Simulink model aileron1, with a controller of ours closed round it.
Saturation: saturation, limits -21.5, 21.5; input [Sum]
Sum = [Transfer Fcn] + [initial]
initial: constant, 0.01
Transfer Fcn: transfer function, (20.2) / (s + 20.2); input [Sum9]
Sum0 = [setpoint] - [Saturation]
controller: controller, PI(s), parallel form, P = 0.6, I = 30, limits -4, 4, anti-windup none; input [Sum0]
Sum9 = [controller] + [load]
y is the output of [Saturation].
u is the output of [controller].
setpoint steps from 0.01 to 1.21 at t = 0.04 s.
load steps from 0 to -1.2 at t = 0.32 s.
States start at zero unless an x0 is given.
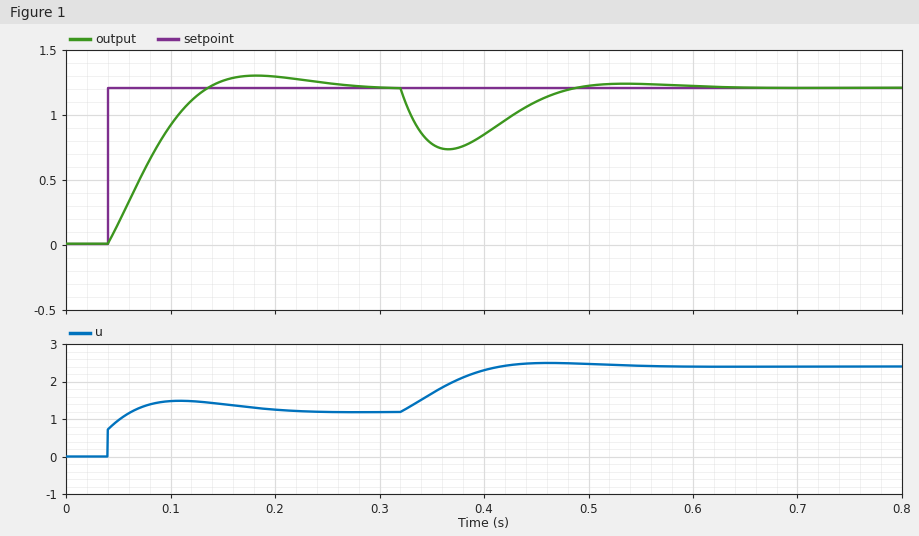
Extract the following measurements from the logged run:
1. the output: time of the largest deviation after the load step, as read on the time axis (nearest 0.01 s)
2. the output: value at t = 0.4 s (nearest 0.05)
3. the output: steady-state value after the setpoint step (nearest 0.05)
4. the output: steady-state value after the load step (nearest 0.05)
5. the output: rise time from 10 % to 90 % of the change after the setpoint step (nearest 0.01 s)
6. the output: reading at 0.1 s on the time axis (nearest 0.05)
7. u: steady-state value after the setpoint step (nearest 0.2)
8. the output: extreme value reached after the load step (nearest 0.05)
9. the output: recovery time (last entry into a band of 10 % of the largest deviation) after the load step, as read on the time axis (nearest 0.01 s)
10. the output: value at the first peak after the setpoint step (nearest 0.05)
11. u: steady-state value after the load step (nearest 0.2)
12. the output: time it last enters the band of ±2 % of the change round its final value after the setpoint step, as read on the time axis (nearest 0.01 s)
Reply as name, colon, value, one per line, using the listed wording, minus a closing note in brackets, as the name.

the output: time of the largest deviation after the load step, as read on the time axis: 0.37 s
the output: value at t = 0.4 s: 0.85
the output: steady-state value after the setpoint step: 1.20
the output: steady-state value after the load step: 1.20
the output: rise time from 10 % to 90 % of the change after the setpoint step: 0.07 s
the output: reading at 0.1 s on the time axis: 0.90
u: steady-state value after the setpoint step: 1.2
the output: extreme value reached after the load step: 0.75
the output: recovery time (last entry into a band of 10 % of the largest deviation) after the load step, as read on the time axis: 0.47 s
the output: value at the first peak after the setpoint step: 1.30
u: steady-state value after the load step: 2.4
the output: time it last enters the band of ±2 % of the change round its final value after the setpoint step, as read on the time axis: 0.26 s
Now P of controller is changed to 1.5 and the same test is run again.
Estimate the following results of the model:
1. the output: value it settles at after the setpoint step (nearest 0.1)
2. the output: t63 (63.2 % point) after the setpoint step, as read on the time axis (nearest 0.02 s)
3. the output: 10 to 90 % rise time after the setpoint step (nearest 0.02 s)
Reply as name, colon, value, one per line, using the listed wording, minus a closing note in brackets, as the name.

the output: value it settles at after the setpoint step: 1.2
the output: t63 (63.2 % point) after the setpoint step, as read on the time axis: 0.08 s
the output: 10 to 90 % rise time after the setpoint step: 0.08 s
